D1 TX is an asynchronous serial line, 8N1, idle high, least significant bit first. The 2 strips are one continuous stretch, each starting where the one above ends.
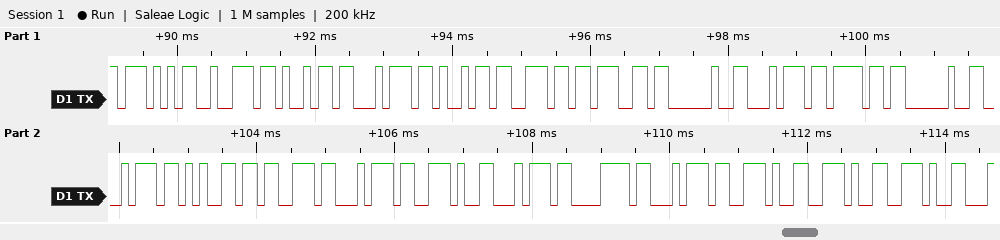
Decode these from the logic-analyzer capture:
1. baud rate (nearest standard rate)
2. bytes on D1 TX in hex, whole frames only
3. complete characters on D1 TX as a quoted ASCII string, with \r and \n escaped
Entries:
9600 baud
57 72 69 74 69 6E 67 20 74 6F 20 74 65 73 74 2E 74 78 74 2E 2E 2E
"Writing to test.txt..."
